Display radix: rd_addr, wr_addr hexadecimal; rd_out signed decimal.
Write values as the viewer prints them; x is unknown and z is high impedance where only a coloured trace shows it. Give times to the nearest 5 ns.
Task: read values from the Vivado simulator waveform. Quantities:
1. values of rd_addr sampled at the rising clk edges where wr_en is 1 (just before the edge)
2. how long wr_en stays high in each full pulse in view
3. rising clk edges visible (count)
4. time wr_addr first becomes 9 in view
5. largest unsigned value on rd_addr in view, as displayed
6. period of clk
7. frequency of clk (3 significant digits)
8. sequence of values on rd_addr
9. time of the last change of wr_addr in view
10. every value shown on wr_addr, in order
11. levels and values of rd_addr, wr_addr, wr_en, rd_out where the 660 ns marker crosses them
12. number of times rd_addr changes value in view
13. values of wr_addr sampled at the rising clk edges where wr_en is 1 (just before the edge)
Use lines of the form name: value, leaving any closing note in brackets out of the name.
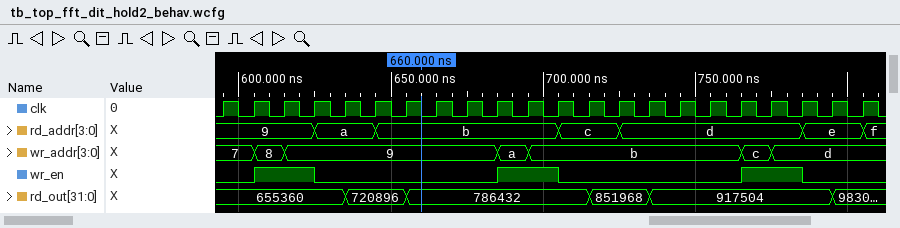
values of rd_addr sampled at the rising clk edges where wr_en is 1: 9, 9, b, b, d, d
how long wr_en stays high in each full pulse in view: 20 ns, 20 ns, 20 ns
rising clk edges visible: 22
time wr_addr first becomes 9 in view: 615 ns
largest unsigned value on rd_addr in view, as displayed: f
period of clk: 10 ns
frequency of clk: 100 MHz
sequence of values on rd_addr: 9, a, b, c, d, e, f
time of the last change of wr_addr in view: 775 ns
every value shown on wr_addr, in order: 7, 8, 9, a, b, c, d
levels and values of rd_addr, wr_addr, wr_en, rd_out where the 660 ns marker crosses them: rd_addr=b, wr_addr=9, wr_en=0, rd_out=786432
number of times rd_addr changes value in view: 6
values of wr_addr sampled at the rising clk edges where wr_en is 1: 8, 9, a, b, c, d
